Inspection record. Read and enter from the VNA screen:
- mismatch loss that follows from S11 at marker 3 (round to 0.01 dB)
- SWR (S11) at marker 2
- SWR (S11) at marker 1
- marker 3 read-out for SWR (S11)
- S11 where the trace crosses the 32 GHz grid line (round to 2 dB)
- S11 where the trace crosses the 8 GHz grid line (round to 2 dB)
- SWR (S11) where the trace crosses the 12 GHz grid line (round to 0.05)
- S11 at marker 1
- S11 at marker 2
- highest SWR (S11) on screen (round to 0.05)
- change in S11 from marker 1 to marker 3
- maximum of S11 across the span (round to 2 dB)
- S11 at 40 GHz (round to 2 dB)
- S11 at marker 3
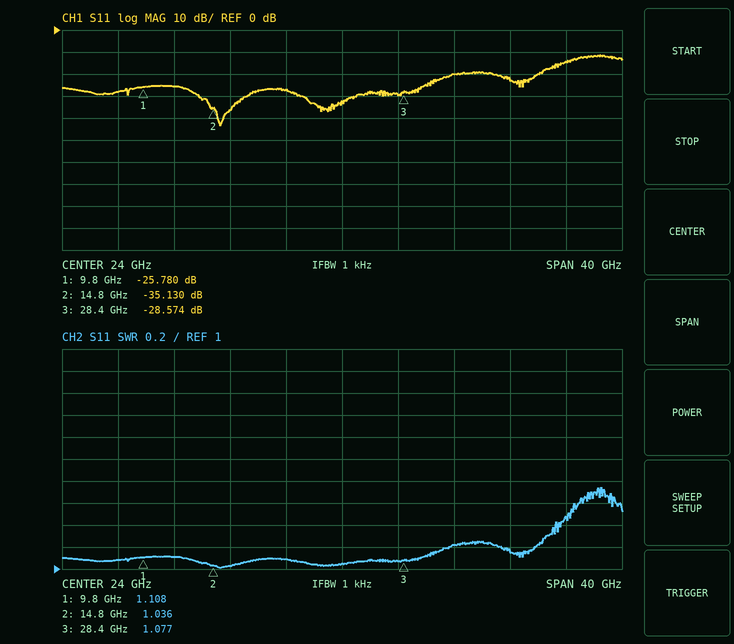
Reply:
0.01 dB
1.036
1.108
1.077
-20 dB
-28 dB
1.10
-25.780 dB
-35.130 dB
1.75
-2.794 dB
-12 dB
-14 dB
-28.574 dB
